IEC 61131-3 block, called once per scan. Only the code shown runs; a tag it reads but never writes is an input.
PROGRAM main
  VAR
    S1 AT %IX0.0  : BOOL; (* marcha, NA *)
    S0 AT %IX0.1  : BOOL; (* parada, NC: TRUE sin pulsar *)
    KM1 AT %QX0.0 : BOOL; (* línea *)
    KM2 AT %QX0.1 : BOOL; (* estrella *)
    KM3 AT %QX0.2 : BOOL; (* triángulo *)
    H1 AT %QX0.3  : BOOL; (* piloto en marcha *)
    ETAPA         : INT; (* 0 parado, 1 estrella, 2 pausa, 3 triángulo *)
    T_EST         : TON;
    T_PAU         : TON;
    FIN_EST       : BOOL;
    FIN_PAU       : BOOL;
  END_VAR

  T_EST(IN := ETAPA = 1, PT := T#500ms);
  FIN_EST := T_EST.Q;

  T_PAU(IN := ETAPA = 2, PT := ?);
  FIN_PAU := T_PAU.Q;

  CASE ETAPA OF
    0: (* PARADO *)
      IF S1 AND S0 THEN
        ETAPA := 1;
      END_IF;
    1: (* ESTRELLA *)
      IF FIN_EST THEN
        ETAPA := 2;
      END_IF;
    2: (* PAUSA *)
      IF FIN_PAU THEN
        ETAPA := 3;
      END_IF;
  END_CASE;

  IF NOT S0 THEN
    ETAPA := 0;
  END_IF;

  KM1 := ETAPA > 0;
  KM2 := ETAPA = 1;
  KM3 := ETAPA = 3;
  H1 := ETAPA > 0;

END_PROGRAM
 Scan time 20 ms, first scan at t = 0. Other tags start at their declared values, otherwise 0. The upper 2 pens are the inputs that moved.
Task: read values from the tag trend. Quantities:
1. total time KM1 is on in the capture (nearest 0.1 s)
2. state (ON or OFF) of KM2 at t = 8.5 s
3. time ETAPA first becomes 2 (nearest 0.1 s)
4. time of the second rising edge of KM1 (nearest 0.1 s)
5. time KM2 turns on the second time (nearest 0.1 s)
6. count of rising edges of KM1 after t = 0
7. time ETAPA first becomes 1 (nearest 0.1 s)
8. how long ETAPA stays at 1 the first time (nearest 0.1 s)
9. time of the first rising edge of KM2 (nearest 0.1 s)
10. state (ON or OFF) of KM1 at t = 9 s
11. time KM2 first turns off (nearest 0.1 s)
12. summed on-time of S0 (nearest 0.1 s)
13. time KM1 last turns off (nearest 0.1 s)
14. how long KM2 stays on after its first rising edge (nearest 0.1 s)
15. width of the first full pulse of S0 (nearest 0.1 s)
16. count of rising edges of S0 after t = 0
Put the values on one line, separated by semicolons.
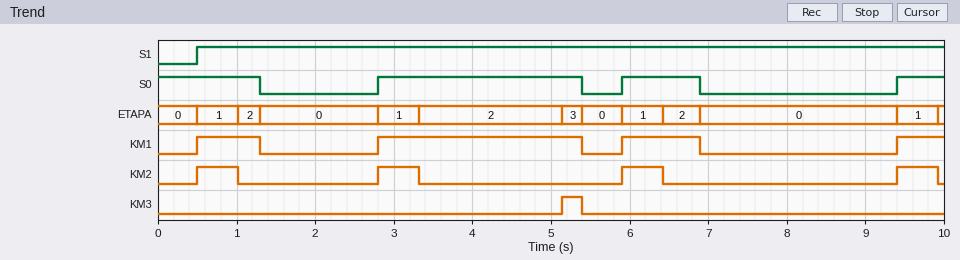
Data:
5.0 s; OFF; 1.0 s; 2.8 s; 2.8 s; 4; 0.5 s; 0.5 s; 0.5 s; OFF; 1.0 s; 5.5 s; 6.9 s; 0.5 s; 2.6 s; 3
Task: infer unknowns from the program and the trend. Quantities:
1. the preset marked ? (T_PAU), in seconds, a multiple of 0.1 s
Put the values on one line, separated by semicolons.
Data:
1.8 s
